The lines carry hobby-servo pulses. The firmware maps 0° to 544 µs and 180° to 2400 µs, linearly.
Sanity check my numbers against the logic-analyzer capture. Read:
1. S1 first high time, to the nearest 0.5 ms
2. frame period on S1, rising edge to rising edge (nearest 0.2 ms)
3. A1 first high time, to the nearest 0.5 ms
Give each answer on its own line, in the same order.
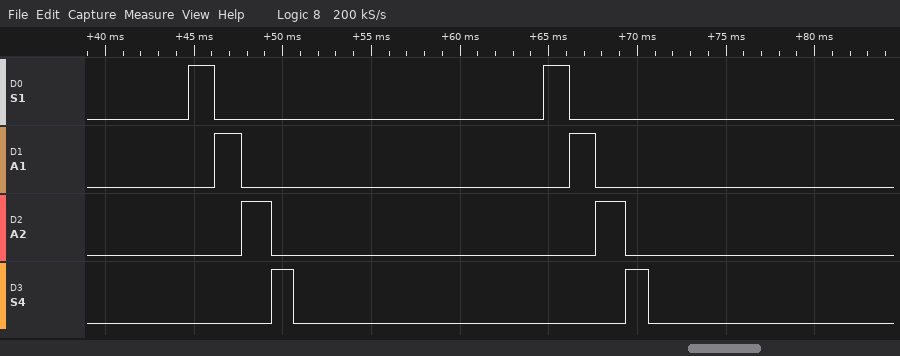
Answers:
1.5 ms
20.0 ms
1.5 ms
